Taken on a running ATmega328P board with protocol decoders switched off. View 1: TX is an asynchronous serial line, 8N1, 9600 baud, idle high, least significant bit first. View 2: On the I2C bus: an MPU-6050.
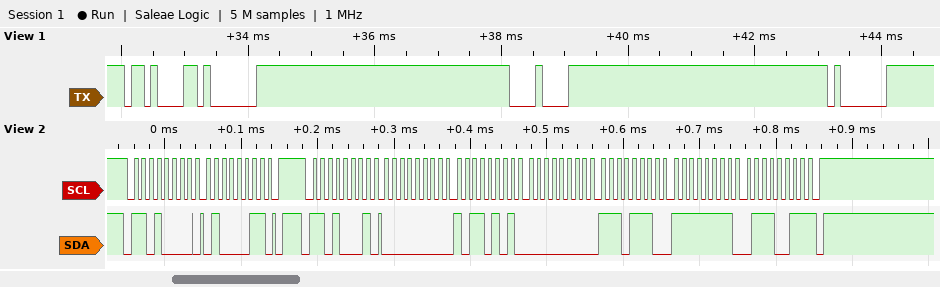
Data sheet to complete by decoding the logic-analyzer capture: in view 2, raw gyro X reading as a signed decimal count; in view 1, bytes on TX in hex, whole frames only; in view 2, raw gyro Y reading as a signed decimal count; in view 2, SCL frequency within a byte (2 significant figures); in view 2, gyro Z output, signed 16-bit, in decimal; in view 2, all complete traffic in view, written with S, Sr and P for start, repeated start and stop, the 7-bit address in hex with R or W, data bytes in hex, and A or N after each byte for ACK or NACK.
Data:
181
0B 01 08 01
238
100 kHz
-141
S 68W A 43 A P S 68R A 00 A B5 A 00 A EE A FF A 73 N P
